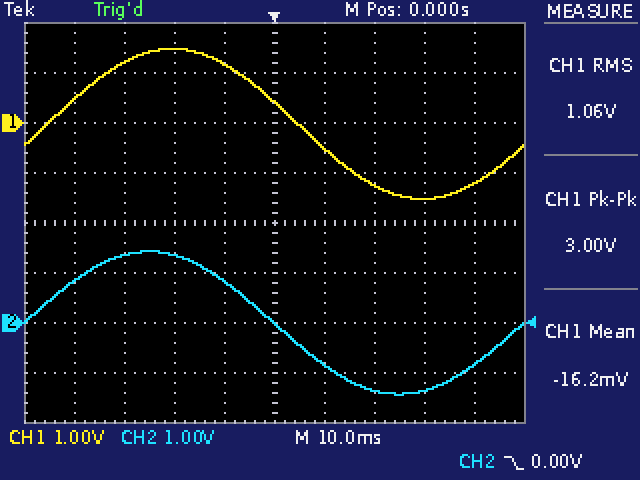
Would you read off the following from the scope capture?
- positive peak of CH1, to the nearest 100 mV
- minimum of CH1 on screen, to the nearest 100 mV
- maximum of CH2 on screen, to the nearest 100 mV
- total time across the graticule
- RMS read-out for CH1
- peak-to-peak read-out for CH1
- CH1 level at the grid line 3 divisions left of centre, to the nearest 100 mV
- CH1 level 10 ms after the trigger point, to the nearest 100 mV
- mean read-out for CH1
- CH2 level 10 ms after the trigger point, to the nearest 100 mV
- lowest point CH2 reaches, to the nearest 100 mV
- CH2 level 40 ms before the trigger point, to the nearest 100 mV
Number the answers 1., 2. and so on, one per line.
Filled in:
1. 1.5 V
2. -1.5 V
3. 1.4 V
4. 100 ms
5. 1.06 V
6. 3.00 V
7. 1.2 V
8. -500 mV
9. -16.2 mV
10. -800 mV
11. -1.4 V
12. 800 mV
